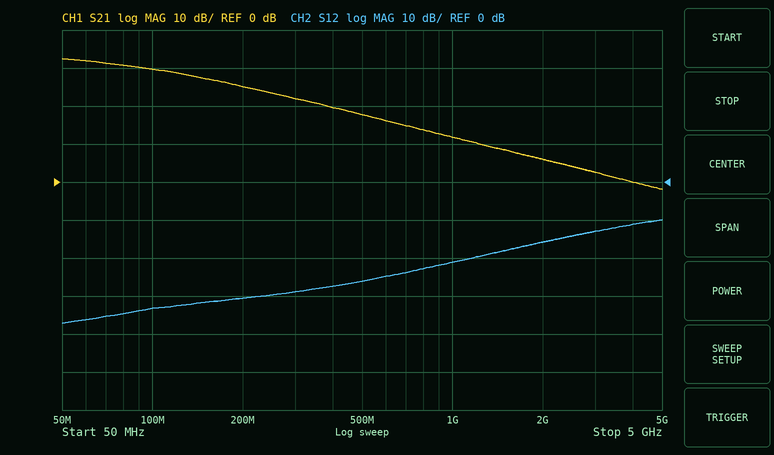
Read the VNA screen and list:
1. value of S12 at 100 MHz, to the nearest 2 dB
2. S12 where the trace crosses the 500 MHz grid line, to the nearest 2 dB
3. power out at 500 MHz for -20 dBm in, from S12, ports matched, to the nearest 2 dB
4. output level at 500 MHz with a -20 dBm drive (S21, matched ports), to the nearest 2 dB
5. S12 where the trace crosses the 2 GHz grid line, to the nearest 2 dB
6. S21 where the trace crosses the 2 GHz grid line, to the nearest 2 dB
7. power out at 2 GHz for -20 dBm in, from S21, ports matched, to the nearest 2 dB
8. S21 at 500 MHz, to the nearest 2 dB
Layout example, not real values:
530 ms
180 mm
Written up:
-34 dB
-26 dB
-46 dBm
-2 dBm
-16 dB
6 dB
-14 dBm
18 dB
